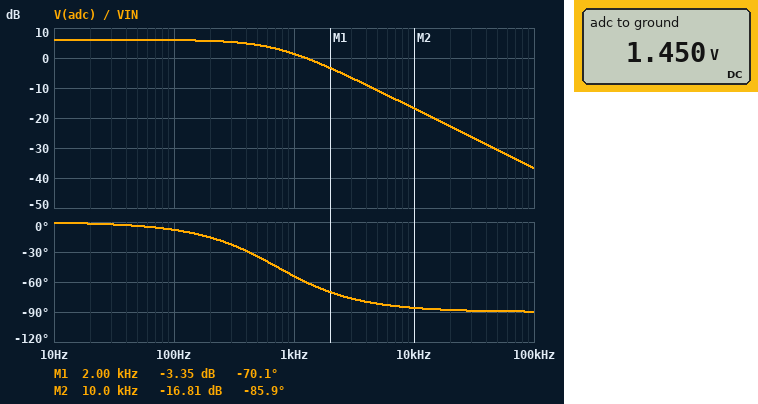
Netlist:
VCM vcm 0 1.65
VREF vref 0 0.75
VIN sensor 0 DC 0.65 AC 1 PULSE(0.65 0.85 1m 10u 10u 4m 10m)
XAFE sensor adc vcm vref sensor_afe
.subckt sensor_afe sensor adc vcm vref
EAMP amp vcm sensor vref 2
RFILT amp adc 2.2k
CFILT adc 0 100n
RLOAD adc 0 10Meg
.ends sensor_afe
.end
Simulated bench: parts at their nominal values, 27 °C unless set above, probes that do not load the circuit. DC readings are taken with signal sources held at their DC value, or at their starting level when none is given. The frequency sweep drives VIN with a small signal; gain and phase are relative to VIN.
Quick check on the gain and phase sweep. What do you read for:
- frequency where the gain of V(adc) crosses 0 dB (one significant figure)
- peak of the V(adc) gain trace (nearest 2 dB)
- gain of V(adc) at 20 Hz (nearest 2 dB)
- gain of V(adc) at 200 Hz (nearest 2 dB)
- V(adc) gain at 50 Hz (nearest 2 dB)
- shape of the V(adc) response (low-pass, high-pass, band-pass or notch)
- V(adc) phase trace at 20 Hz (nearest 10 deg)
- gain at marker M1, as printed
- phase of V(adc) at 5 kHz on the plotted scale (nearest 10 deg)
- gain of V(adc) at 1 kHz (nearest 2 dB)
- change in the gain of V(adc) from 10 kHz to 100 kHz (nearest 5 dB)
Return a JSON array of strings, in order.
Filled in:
["1 kHz", "6 dB", "6 dB", "6 dB", "6 dB", "low-pass", "0 deg", "-3.35 dB", "-80 deg", "2 dB", "-20 dB"]
